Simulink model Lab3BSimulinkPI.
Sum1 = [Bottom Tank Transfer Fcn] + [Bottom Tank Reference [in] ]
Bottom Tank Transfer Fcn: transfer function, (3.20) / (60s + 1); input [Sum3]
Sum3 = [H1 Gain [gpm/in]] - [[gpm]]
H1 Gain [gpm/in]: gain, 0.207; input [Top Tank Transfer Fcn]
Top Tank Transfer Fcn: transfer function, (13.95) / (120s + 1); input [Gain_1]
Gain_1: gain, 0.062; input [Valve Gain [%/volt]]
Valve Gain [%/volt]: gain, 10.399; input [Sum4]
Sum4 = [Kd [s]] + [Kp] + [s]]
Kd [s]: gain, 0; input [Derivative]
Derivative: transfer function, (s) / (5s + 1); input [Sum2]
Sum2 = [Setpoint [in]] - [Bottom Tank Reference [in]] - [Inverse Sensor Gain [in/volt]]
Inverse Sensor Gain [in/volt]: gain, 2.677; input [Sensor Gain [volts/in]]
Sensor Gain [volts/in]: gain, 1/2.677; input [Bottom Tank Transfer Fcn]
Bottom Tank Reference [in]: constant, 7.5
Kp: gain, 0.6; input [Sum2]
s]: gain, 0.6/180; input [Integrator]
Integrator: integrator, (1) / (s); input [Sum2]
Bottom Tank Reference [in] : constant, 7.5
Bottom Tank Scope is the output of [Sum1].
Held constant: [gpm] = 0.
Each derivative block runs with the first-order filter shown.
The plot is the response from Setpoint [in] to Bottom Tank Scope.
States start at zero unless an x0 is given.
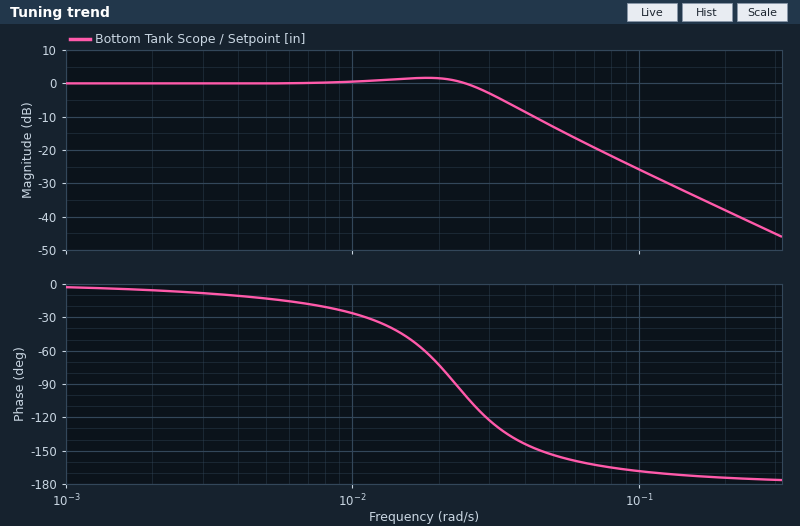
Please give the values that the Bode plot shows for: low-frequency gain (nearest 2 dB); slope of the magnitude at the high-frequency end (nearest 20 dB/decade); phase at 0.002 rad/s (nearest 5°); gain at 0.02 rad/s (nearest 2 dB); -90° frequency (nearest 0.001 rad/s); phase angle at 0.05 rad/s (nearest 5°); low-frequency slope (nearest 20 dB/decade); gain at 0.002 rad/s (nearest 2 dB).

0 dB
-40 dB/decade
-5°
2 dB
0.023 rad/s
-155°
0 dB/decade
0 dB
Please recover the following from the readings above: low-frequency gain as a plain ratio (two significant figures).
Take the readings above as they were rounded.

1.0
